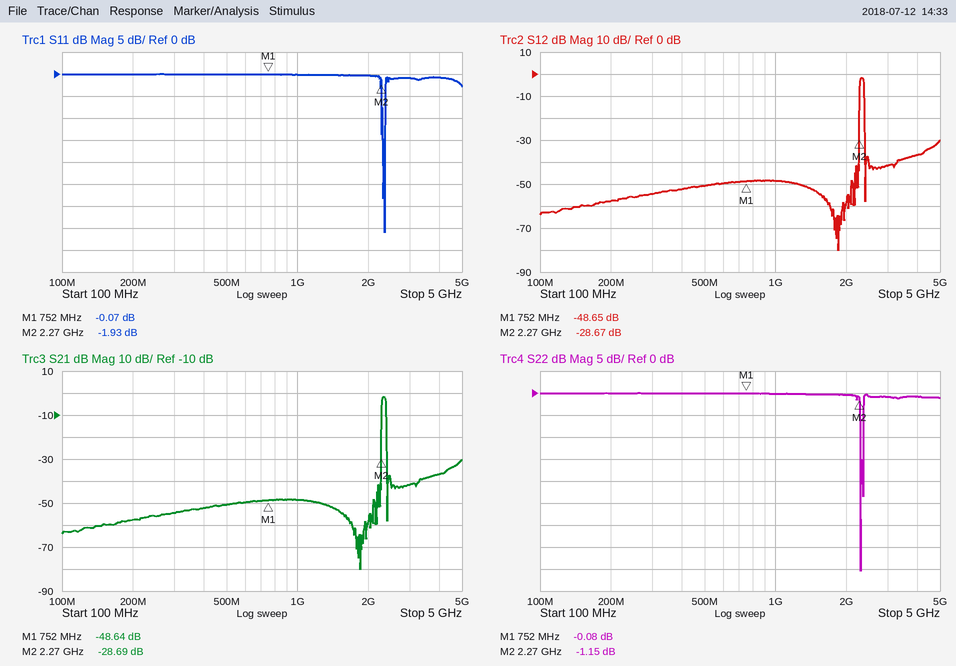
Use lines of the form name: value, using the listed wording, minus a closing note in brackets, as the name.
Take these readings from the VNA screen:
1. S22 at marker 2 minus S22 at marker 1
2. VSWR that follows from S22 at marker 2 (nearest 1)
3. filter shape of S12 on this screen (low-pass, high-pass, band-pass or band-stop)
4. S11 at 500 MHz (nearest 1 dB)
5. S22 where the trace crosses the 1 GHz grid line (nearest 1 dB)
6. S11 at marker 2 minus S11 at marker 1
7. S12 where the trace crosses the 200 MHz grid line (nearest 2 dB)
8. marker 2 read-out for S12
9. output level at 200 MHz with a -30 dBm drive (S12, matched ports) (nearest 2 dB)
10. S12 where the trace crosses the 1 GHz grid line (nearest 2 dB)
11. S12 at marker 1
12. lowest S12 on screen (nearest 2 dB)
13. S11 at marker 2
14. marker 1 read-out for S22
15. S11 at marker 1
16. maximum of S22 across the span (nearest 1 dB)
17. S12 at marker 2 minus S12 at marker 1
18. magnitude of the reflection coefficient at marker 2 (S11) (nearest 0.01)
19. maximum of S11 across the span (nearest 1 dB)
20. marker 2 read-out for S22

S22 at marker 2 minus S22 at marker 1: -1.07 dB
VSWR that follows from S22 at marker 2: 15
filter shape of S12 on this screen: band-pass
S11 at 500 MHz: 0 dB
S22 where the trace crosses the 1 GHz grid line: 0 dB
S11 at marker 2 minus S11 at marker 1: -1.86 dB
S12 where the trace crosses the 200 MHz grid line: -58 dB
marker 2 read-out for S12: -28.67 dB
output level at 200 MHz with a -30 dBm drive (S12, matched ports): -88 dBm
S12 where the trace crosses the 1 GHz grid line: -48 dB
S12 at marker 1: -48.65 dB
lowest S12 on screen: -80 dB
S11 at marker 2: -1.93 dB
marker 1 read-out for S22: -0.08 dB
S11 at marker 1: -0.07 dB
maximum of S22 across the span: 0 dB
S12 at marker 2 minus S12 at marker 1: 19.98 dB
magnitude of the reflection coefficient at marker 2 (S11): 0.80
maximum of S11 across the span: 0 dB
marker 2 read-out for S22: -1.15 dB
